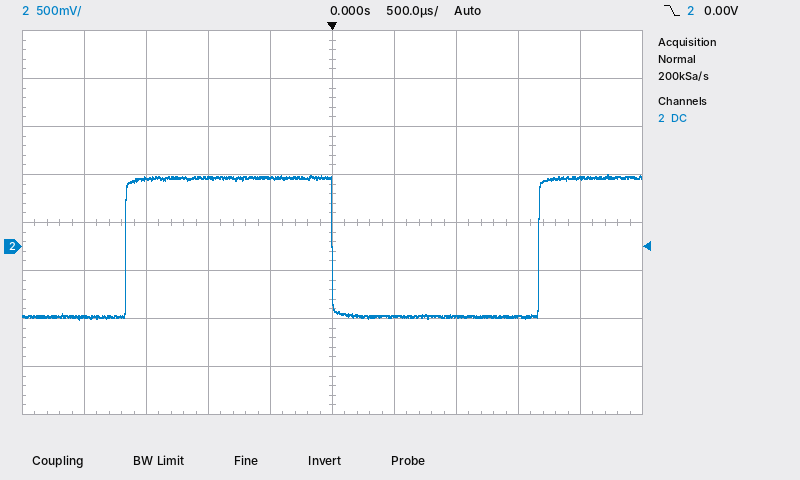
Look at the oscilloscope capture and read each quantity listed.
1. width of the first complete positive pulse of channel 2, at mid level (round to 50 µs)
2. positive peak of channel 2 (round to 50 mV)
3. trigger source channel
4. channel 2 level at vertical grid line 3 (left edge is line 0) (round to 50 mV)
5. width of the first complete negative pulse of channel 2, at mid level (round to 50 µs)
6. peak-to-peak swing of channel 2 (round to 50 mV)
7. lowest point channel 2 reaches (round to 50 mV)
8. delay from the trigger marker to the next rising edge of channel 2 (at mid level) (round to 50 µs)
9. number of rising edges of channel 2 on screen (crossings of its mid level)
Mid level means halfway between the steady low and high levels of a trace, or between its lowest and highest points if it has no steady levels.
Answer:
1.65 ms
750 mV
channel 2
700 mV
1.65 ms
1.50 V
-750 mV
1.65 ms
2
